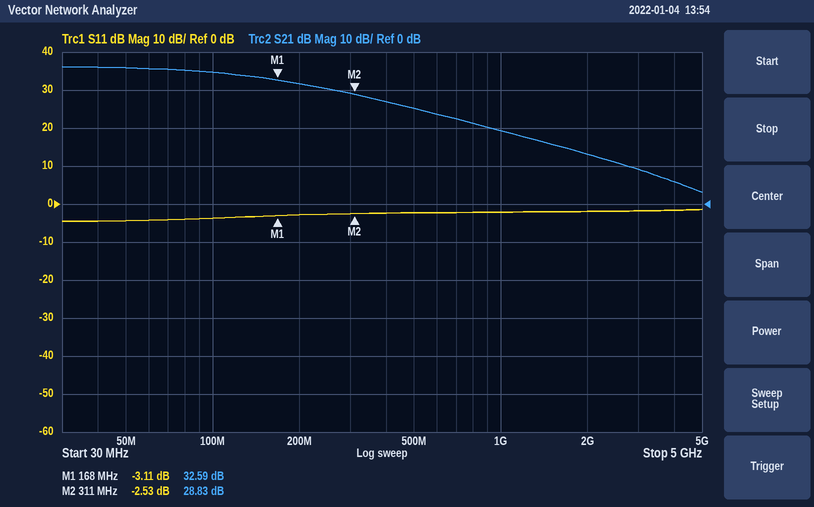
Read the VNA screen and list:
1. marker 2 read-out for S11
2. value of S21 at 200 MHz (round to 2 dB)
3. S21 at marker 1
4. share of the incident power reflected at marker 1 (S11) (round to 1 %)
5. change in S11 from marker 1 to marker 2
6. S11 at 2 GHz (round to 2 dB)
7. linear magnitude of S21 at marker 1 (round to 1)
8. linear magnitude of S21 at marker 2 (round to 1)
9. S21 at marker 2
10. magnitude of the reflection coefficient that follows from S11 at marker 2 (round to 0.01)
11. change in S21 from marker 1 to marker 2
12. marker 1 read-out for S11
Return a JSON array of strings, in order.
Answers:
["-2.53 dB", "32 dB", "32.59 dB", "49 %", "0.58 dB", "-2 dB", "43", "28", "28.83 dB", "0.75", "-3.76 dB", "-3.11 dB"]
